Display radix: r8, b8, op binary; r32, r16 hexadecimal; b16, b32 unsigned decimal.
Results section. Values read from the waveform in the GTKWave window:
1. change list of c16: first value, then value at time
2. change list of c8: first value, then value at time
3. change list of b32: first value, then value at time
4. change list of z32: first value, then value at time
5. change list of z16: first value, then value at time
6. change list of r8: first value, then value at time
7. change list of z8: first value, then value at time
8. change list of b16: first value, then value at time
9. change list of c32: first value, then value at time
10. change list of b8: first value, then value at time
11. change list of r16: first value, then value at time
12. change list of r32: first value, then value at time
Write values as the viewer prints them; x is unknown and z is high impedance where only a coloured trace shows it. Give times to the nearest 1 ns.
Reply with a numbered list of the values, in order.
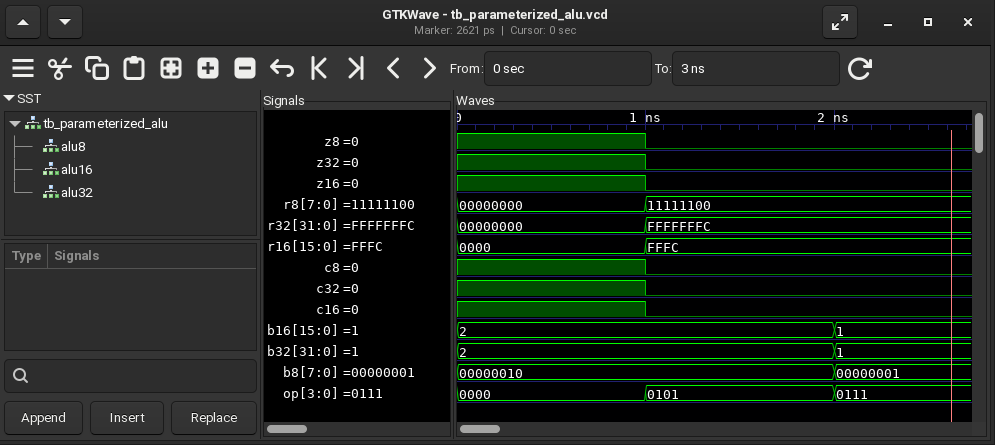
1. 1, 0 at 1 ns
2. 1, 0 at 1 ns
3. 2, 1 at 2 ns
4. 1, 0 at 1 ns
5. 1, 0 at 1 ns
6. 00000000, 11111100 at 1 ns
7. 1, 0 at 1 ns
8. 2, 1 at 2 ns
9. 1, 0 at 1 ns
10. 00000010, 00000001 at 2 ns
11. 0000, FFFC at 1 ns
12. 00000000, FFFFFFFC at 1 ns
